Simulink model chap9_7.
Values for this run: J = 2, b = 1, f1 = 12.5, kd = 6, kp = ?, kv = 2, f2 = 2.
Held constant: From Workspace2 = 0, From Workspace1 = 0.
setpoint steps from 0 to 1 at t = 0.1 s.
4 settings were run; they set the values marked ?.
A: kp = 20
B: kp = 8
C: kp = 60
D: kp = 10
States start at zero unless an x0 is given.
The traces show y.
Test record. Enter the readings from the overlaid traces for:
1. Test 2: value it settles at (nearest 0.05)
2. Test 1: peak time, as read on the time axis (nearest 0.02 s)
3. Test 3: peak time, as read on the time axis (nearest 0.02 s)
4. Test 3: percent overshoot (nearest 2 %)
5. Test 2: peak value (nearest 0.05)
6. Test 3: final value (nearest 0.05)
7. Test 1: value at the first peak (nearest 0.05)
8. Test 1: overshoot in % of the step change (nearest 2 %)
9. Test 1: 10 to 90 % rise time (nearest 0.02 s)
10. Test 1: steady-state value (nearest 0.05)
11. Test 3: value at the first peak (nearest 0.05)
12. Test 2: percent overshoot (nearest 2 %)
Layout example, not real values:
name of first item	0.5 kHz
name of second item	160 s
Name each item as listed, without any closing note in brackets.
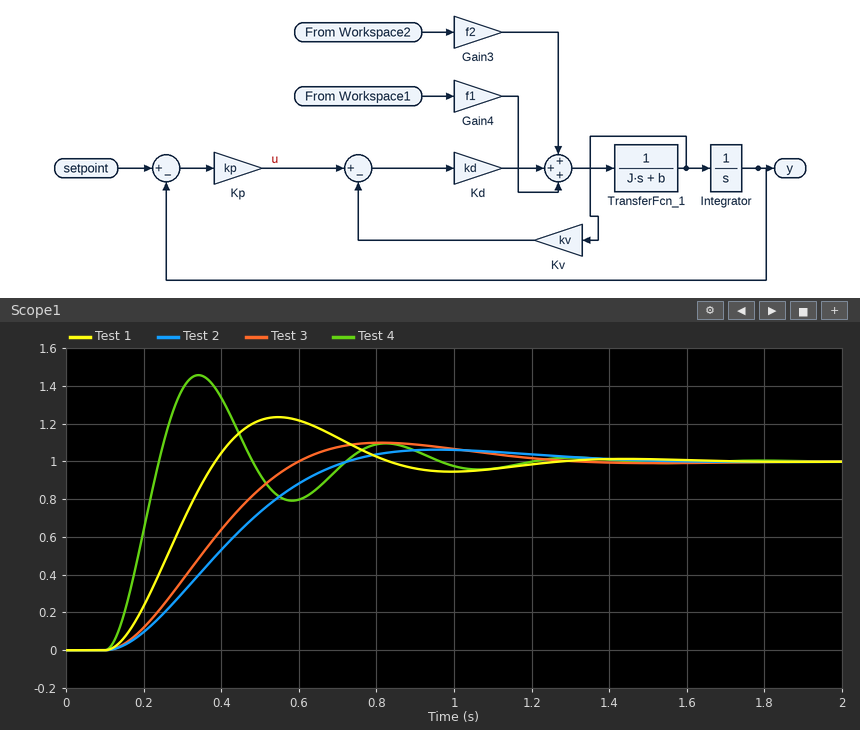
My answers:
Test 2: value it settles at	1.00
Test 1: peak time, as read on the time axis	0.54 s
Test 3: peak time, as read on the time axis	0.82 s
Test 3: percent overshoot	10 %
Test 2: peak value	1.05
Test 3: final value	1.00
Test 1: value at the first peak	1.25
Test 1: overshoot in % of the step change	24 %
Test 1: 10 to 90 % rise time	0.20 s
Test 1: steady-state value	1.00
Test 3: value at the first peak	1.10
Test 2: percent overshoot	6 %
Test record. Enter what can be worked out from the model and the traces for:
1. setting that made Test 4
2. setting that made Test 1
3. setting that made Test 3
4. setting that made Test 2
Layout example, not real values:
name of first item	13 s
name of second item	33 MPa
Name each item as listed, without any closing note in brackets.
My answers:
setting that made Test 4	C
setting that made Test 1	A
setting that made Test 3	D
setting that made Test 2	B
